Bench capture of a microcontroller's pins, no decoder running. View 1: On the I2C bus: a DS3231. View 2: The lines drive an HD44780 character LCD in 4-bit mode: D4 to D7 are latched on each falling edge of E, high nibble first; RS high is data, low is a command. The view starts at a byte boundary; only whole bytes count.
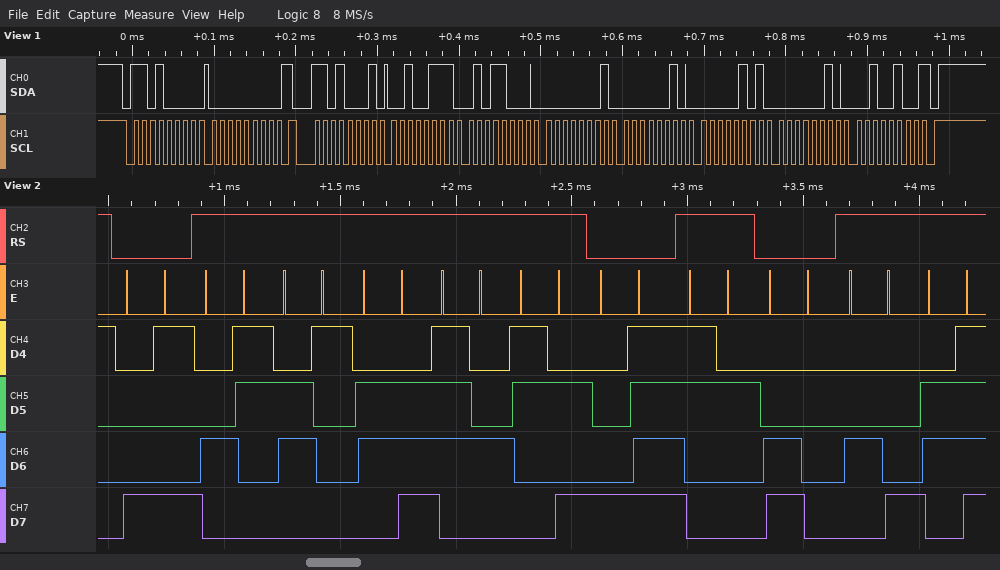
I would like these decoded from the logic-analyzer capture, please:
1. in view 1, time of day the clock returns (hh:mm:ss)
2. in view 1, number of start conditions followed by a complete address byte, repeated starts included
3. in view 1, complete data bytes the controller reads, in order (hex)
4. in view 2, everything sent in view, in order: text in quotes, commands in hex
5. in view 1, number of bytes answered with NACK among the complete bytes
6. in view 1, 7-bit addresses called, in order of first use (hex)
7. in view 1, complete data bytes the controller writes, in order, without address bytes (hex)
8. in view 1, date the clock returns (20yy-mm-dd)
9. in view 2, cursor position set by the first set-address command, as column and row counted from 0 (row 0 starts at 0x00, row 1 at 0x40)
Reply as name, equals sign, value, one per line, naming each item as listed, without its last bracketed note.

in view 1, time of day the clock returns = 01:58:27
in view 1, number of start conditions followed by a complete address byte, repeated starts included = 2
in view 1, complete data bytes the controller reads, in order = 27 58 01 02 05 02 24
in view 2, everything sent in view, in order: text in quotes, commands in hex = 0x89 "Cant:" 0x8F "2" 0xC0 "Ho"
in view 1, number of bytes answered with NACK among the complete bytes = 1
in view 1, 7-bit addresses called, in order of first use = 0x68
in view 1, complete data bytes the controller writes, in order, without address bytes = 00
in view 1, date the clock returns = 2024-02-05
in view 2, cursor position set by the first set-address command, as column and row counted from 0 = column 9, row 0
